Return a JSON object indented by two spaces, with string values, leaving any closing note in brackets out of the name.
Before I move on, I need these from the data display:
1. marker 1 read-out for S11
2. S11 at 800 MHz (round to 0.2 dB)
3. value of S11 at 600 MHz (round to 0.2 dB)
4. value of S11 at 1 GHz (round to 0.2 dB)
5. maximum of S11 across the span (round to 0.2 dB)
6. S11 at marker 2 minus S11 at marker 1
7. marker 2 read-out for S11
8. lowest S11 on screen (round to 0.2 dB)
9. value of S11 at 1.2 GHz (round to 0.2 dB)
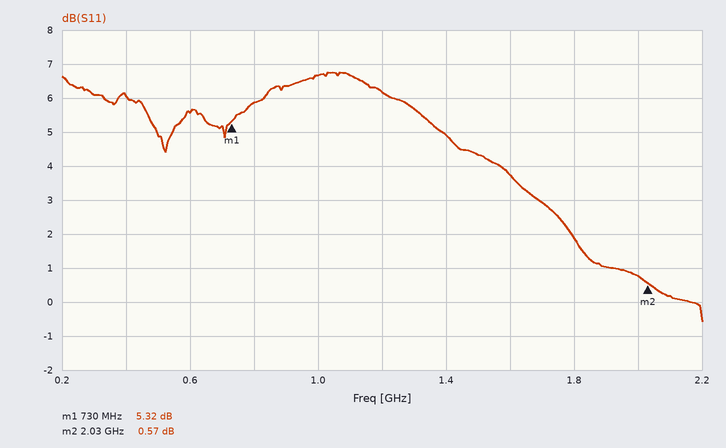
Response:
{
  "marker 1 read-out for S11": "5.32 dB",
  "S11 at 800 MHz": "5.8 dB",
  "value of S11 at 600 MHz": "5.6 dB",
  "value of S11 at 1 GHz": "6.6 dB",
  "maximum of S11 across the span": "6.8 dB",
  "S11 at marker 2 minus S11 at marker 1": "-4.75 dB",
  "marker 2 read-out for S11": "0.57 dB",
  "lowest S11 on screen": "-0.6 dB",
  "value of S11 at 1.2 GHz": "6.2 dB"
}
